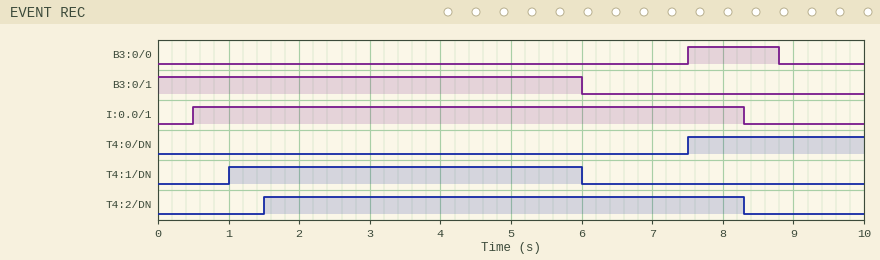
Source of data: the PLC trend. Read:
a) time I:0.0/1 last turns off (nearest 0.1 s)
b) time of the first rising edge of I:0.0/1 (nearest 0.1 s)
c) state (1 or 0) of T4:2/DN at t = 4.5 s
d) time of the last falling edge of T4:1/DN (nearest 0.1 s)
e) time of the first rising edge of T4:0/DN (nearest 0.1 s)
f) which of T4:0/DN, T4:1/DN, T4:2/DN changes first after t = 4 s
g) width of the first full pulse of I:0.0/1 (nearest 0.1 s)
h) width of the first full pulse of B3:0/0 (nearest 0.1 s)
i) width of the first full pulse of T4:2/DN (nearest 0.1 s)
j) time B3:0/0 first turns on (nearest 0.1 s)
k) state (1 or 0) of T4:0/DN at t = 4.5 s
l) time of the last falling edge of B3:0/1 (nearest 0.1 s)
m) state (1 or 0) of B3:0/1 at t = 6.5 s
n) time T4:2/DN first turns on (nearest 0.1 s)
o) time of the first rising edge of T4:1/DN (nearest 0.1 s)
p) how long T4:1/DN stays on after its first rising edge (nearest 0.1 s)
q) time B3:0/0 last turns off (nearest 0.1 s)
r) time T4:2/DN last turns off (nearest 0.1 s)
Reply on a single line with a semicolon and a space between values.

8.3 s; 0.5 s; 1; 6.0 s; 7.5 s; T4:1/DN; 7.8 s; 1.3 s; 6.8 s; 7.5 s; 0; 6.0 s; 0; 1.5 s; 1.0 s; 5.0 s; 8.8 s; 8.3 s
